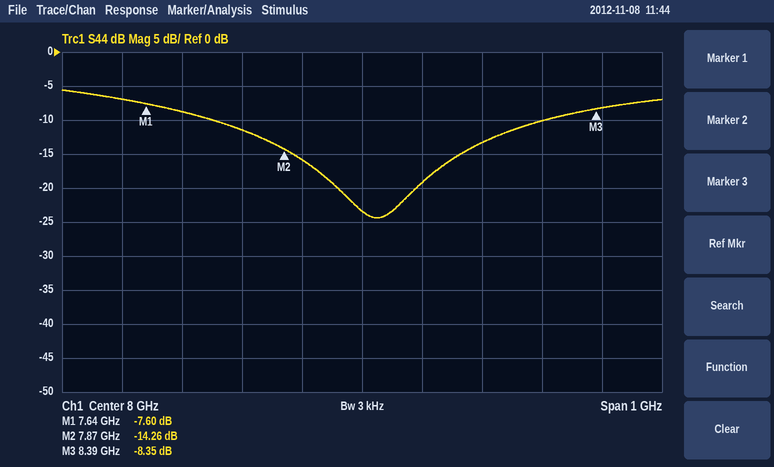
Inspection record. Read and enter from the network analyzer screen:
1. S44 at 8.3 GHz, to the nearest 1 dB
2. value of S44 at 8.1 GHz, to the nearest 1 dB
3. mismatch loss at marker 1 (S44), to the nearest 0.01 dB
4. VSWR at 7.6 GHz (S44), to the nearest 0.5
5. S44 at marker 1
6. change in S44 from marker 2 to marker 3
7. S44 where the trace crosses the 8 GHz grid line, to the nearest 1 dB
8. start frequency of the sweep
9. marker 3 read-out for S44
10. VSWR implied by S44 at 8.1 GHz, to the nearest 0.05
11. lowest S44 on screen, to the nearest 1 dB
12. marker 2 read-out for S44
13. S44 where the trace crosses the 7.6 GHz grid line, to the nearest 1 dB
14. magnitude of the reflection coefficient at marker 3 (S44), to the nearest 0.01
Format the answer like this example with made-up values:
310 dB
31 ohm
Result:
-10 dB
-19 dB
0.83 dB
2.5
-7.60 dB
5.91 dB
-23 dB
7.5 GHz
-8.35 dB
1.25
-24 dB
-14.26 dB
-7 dB
0.38
